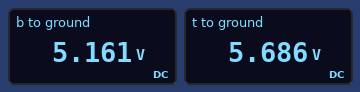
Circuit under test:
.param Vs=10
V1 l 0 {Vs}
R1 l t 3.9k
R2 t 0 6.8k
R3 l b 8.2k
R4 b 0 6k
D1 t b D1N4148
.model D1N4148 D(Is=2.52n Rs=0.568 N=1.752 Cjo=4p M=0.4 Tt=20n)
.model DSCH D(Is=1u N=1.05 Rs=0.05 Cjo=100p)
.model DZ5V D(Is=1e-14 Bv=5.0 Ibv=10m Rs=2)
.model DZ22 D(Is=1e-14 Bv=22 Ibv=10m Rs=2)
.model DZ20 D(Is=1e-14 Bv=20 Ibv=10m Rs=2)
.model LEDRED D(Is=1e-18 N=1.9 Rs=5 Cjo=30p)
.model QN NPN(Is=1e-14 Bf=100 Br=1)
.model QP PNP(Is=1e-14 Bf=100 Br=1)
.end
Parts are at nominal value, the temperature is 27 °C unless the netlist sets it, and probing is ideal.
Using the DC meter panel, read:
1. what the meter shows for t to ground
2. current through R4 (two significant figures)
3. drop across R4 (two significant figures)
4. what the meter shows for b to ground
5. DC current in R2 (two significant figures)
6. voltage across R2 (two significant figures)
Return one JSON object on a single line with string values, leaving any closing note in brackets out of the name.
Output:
{"what the meter shows for t to ground": "5.686 V", "current through R4": "860 µA", "drop across R4": "5.2 V", "what the meter shows for b to ground": "5.161 V", "DC current in R2": "840 µA", "voltage across R2": "5.7 V"}
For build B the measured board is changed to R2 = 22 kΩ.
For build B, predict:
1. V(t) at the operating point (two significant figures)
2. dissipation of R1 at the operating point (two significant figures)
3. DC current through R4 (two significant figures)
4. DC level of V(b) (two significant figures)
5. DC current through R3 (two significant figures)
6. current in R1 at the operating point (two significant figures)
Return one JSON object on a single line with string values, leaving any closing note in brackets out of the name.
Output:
{"V(t) at the operating point": "6.7 V", "dissipation of R1 at the operating point": "2.8 mW", "DC current through R4": "1.0 mA", "DC level of V(b)": "6.1 V", "DC current through R3": "470 µA", "current in R1 at the operating point": "850 µA"}
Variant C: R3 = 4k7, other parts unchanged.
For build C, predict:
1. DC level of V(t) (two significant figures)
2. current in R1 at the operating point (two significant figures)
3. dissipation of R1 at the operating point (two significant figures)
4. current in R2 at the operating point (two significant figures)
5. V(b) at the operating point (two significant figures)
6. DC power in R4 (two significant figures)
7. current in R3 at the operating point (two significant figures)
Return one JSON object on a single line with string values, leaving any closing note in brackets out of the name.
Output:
{"DC level of V(t)": "6.2 V", "current in R1 at the operating point": "970 µA", "dissipation of R1 at the operating point": "3.7 mW", "current in R2 at the operating point": "910 µA", "V(b) at the operating point": "5.8 V", "DC power in R4": "5.5 mW", "current in R3 at the operating point": "900 µA"}
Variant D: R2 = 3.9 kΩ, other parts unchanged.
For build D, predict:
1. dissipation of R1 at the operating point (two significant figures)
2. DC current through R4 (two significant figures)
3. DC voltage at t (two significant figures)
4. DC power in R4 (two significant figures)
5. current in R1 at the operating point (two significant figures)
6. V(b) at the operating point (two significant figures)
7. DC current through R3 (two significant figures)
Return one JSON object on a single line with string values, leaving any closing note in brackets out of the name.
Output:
{"dissipation of R1 at the operating point": "6.7 mW", "DC current through R4": "740 µA", "DC voltage at t": "4.9 V", "DC power in R4": "3.3 mW", "current in R1 at the operating point": "1.3 mA", "V(b) at the operating point": "4.4 V", "DC current through R3": "680 µA"}
